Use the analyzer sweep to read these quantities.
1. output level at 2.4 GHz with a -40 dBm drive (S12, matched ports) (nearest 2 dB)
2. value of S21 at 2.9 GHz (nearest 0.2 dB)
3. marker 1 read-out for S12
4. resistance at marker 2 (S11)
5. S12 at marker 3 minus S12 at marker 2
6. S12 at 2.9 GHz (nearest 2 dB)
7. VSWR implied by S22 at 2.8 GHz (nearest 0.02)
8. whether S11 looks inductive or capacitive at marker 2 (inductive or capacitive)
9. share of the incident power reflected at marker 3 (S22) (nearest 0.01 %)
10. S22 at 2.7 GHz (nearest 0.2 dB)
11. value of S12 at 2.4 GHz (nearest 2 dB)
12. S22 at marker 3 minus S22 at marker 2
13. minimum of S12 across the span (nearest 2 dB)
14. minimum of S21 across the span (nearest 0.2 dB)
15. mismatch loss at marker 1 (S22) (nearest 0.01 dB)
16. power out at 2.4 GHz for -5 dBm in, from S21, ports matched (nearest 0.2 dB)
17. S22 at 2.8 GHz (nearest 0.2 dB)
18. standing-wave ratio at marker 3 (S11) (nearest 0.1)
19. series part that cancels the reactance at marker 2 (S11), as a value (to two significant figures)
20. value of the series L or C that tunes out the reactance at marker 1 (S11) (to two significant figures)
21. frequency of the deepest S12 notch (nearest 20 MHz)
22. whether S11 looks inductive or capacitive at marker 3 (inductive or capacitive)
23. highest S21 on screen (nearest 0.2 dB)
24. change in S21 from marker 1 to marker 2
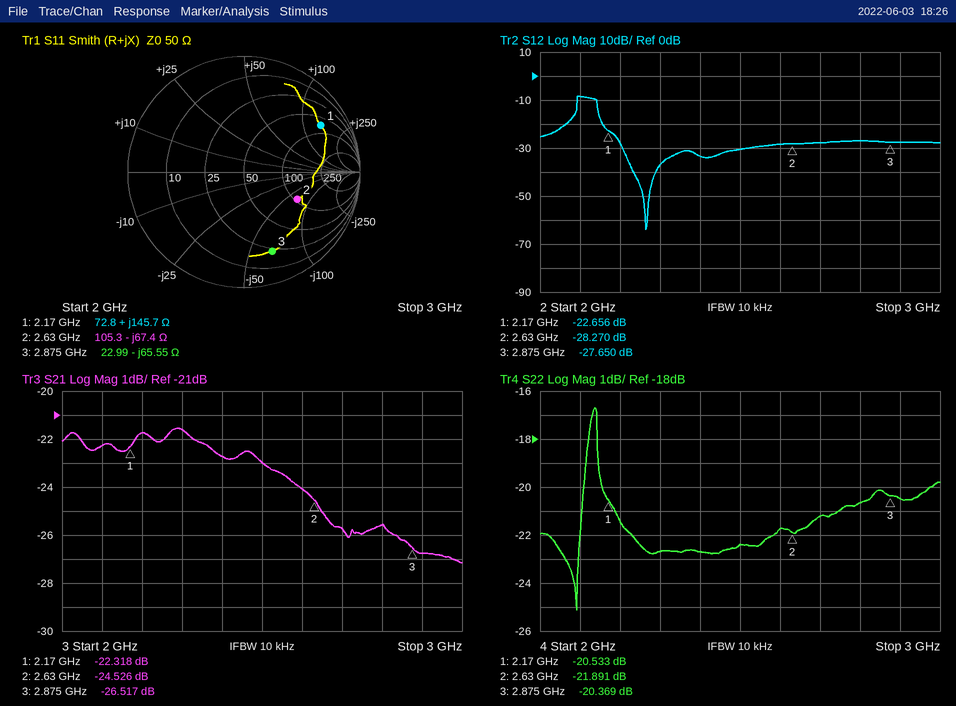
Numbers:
-74 dBm
-26.8 dB
-22.656 dB
105.3 Ω
0.620 dB
-28 dB
1.20
capacitive
0.92 %
-21.2 dB
-34 dB
1.522 dB
-64 dB
-27.2 dB
0.04 dB
-27.8 dBm
-20.6 dB
6.2
4.1 nH
500 fF
2.26 GHz
capacitive
-21.6 dB
-2.208 dB
